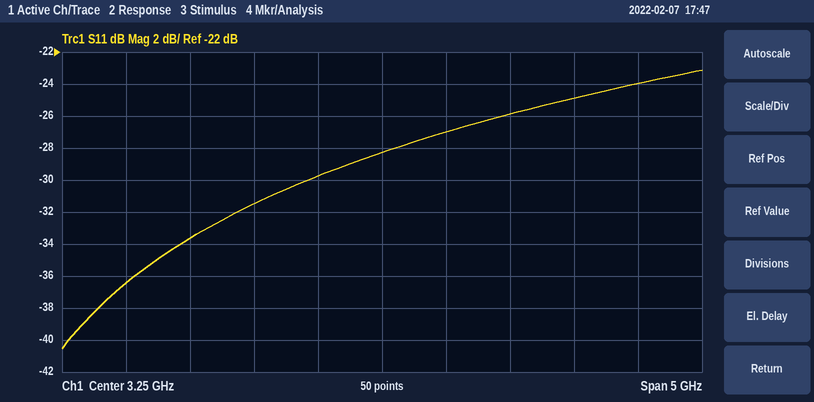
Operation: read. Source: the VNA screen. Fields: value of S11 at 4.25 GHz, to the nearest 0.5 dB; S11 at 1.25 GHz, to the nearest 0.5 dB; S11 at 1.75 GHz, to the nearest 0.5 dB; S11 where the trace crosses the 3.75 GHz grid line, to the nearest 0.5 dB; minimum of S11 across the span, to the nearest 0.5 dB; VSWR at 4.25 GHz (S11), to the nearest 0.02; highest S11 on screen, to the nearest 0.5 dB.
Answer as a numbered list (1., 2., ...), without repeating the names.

1. -26.0 dB
2. -36.5 dB
3. -33.5 dB
4. -27.0 dB
5. -40.5 dB
6. 1.10
7. -23.0 dB
